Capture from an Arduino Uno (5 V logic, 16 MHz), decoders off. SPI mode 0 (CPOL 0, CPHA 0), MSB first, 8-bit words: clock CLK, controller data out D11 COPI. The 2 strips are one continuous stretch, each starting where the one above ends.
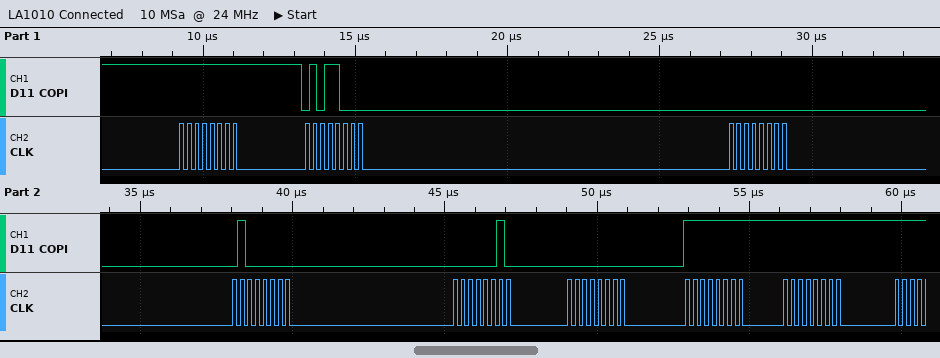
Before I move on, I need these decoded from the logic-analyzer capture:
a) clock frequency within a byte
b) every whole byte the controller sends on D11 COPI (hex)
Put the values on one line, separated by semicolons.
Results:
4 MHz; 0xFF 0x58 0x00 0x40 0x02 0x00 0xFF 0xFF
